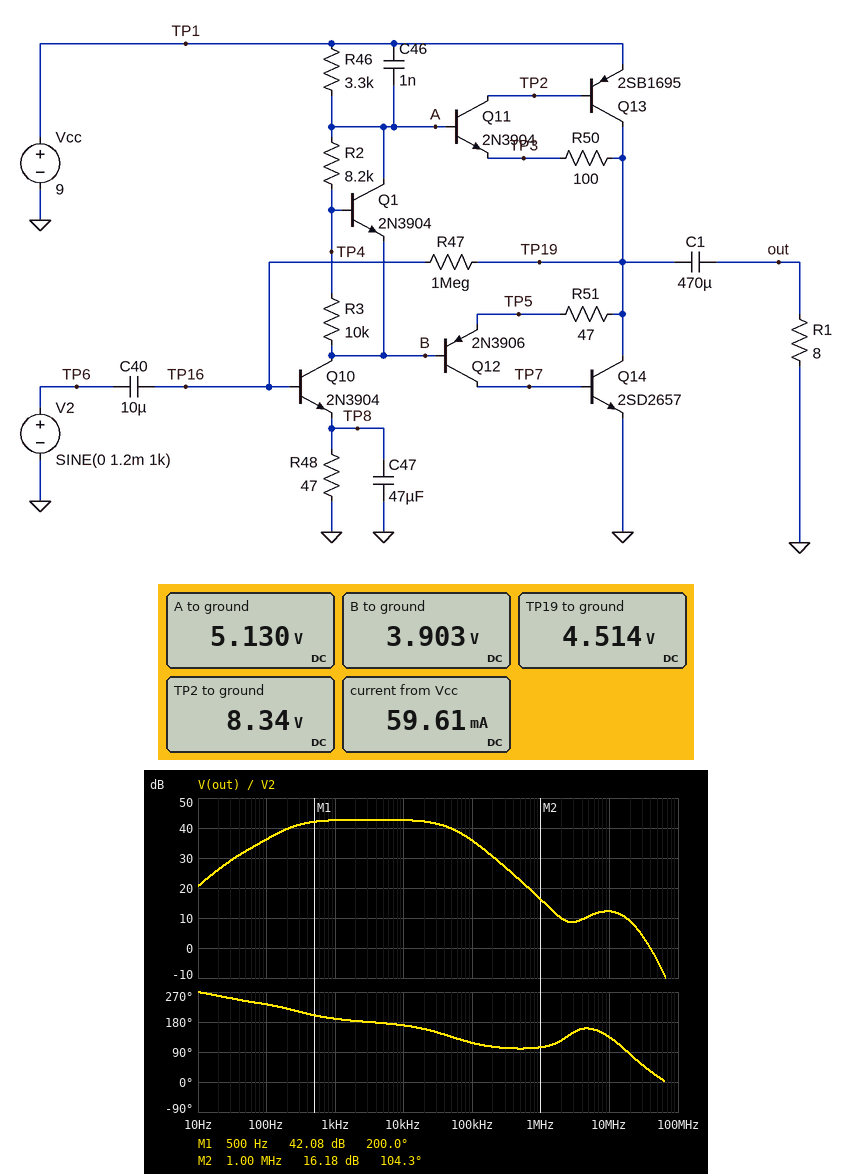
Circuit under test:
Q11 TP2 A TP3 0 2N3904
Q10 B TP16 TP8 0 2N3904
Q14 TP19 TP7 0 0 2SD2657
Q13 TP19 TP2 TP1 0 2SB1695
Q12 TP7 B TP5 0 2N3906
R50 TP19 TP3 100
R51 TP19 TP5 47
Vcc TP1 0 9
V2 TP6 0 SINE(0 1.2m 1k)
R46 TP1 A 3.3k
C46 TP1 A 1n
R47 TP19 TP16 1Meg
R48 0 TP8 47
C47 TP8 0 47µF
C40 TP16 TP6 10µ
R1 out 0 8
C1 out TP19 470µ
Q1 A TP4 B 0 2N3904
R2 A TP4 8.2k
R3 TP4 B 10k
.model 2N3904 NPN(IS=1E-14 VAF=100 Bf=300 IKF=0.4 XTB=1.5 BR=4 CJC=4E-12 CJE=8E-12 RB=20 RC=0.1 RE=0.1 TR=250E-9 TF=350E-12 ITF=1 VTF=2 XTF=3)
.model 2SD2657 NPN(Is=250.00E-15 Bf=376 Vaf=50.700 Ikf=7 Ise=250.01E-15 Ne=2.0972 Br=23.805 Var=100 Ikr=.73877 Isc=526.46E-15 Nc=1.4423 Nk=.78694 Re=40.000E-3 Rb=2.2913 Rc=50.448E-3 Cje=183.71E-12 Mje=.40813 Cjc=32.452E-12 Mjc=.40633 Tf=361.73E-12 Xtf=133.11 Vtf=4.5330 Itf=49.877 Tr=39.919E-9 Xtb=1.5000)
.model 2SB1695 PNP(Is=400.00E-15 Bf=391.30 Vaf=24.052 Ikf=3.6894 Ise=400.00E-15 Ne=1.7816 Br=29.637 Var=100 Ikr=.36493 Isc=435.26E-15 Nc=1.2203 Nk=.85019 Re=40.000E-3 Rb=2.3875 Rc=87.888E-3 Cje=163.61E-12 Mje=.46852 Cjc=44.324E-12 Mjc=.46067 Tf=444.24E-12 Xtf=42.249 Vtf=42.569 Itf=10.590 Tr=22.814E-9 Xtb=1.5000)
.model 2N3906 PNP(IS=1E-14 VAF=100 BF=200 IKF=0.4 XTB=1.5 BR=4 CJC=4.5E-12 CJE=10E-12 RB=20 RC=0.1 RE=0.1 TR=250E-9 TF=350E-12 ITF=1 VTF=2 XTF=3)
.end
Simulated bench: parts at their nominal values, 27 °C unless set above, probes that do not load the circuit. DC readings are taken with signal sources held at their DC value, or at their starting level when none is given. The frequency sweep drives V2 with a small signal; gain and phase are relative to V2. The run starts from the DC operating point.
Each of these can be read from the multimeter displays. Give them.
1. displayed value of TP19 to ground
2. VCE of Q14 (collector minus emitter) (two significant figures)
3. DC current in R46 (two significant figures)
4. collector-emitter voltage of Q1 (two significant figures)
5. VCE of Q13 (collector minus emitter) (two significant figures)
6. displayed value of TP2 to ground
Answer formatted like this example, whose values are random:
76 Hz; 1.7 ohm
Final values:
4.514 V; 4.5 V; 1.2 mA; 1.2 V; -4.5 V; 8.34 V
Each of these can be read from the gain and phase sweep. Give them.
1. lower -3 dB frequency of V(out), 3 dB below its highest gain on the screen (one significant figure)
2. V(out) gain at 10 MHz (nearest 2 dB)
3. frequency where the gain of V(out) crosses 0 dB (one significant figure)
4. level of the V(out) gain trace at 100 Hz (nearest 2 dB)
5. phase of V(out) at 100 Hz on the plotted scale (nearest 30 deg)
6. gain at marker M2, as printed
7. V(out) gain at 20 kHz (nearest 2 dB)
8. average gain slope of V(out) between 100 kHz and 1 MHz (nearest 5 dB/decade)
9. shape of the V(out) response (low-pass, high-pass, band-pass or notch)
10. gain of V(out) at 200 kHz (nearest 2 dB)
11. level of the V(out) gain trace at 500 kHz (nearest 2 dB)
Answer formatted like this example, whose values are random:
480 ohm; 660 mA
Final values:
200 Hz; 12 dB; 40 MHz; 36 dB; 240 deg; 16.18 dB; 42 dB; -20 dB/decade; band-pass; 30 dB; 22 dB
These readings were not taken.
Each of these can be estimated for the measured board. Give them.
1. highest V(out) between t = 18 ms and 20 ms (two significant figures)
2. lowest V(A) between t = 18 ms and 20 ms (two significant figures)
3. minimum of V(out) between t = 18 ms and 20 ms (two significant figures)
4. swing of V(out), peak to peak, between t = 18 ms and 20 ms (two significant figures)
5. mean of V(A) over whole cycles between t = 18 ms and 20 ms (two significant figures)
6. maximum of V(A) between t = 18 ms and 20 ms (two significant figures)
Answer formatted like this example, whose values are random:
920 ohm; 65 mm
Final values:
160 mV; 5.0 V; -160 mV; 320 mV; 5.1 V; 5.3 V
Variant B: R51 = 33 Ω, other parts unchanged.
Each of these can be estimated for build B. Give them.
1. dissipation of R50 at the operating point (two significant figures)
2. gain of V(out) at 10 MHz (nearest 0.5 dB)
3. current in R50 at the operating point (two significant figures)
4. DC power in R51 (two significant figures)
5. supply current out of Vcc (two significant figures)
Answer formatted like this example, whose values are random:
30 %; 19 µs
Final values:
1.9 µW; 12.5 dB; 140 µA; 760 nW; 61 mA
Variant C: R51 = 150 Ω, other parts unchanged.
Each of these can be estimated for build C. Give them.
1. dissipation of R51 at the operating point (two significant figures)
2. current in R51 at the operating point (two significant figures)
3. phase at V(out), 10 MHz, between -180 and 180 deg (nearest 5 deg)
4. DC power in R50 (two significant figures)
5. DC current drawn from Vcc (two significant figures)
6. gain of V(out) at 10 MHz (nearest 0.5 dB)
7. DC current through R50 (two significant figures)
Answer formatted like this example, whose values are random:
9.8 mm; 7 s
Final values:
2.3 µW; 120 µA; 120 deg; 1.2 µW; 50 mA; 9.0 dB; 110 µA
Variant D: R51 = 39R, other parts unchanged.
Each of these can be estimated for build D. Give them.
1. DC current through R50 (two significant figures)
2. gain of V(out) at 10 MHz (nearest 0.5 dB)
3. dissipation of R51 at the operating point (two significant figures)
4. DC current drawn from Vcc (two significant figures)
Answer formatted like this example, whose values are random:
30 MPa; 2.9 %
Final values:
140 µA; 12.5 dB; 880 nW; 61 mA
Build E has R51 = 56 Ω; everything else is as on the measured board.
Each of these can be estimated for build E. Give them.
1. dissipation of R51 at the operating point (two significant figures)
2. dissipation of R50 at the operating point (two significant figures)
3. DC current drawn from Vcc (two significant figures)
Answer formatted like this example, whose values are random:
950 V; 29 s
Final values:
1.2 µW; 1.7 µW; 59 mA
